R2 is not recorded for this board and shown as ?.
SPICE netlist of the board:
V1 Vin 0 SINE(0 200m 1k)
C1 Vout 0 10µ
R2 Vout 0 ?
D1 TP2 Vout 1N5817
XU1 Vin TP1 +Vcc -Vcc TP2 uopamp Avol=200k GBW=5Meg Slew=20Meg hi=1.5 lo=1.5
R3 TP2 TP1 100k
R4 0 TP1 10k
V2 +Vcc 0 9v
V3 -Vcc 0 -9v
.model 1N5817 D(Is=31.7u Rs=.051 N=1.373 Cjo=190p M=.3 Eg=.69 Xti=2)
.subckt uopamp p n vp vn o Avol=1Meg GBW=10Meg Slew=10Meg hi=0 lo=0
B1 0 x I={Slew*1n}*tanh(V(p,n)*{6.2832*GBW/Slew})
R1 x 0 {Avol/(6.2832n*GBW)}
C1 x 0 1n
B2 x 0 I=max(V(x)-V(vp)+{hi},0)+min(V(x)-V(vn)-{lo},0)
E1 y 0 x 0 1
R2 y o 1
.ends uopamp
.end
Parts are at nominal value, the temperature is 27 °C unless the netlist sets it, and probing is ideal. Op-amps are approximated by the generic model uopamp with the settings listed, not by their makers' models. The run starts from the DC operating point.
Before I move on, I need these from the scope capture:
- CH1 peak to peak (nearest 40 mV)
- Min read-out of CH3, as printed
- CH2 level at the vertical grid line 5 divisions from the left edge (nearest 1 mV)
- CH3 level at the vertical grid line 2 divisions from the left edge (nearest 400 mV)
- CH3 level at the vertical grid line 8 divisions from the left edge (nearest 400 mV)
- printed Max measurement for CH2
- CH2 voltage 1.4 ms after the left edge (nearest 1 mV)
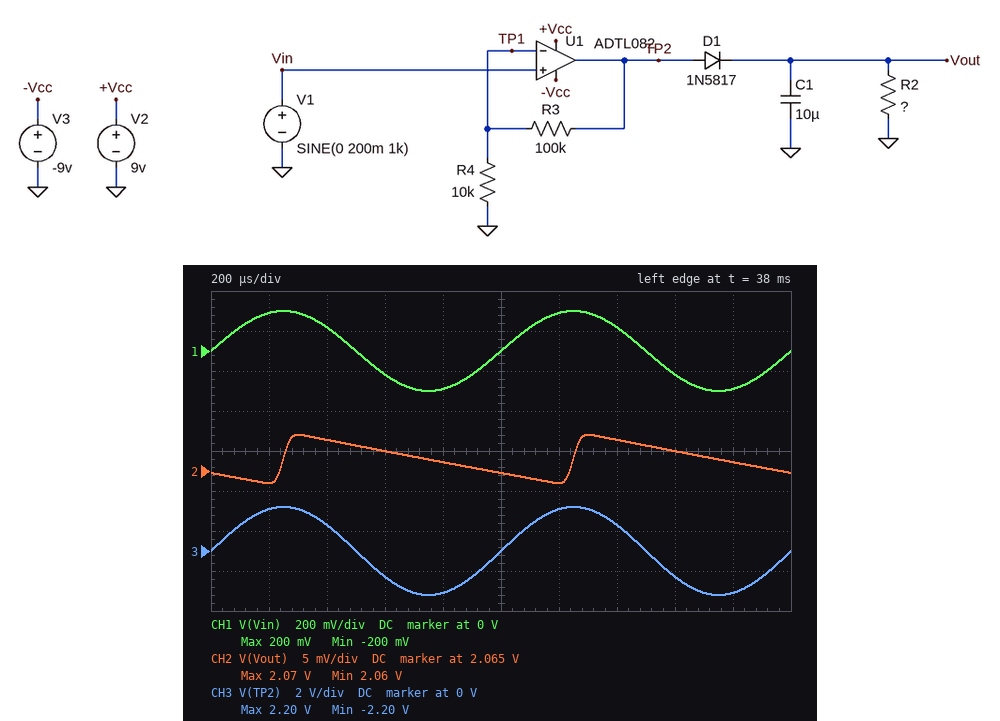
400 mV
-2.20 V
2.065 V
1.2 V
-1.2 V
2.07 V
2.069 V
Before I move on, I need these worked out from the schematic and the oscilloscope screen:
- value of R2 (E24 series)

56 kΩ
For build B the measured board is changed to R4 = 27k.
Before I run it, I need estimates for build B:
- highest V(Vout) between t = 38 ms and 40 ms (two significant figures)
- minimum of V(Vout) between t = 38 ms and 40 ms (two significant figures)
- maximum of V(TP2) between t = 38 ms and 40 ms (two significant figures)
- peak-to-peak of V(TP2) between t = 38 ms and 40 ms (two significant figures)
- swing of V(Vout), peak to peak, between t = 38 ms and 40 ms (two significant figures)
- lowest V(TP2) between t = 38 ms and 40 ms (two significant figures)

840 mV
830 mV
940 mV
1.9 V
3.9 mV
-940 mV
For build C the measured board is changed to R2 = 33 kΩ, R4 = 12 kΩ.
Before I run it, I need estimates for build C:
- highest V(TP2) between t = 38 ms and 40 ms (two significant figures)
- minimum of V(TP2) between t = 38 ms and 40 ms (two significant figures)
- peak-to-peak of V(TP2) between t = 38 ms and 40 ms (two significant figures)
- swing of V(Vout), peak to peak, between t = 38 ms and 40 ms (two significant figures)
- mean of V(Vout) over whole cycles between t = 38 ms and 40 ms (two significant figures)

1.9 V
-1.9 V
3.7 V
7.4 mV
1.7 V
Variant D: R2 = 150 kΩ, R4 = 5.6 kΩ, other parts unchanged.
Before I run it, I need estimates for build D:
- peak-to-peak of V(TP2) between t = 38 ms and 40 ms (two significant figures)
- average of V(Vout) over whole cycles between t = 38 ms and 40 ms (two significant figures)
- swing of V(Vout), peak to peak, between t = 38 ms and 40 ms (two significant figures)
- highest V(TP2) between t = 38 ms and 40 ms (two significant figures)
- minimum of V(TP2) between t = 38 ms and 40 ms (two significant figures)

7.5 V
3.6 V
5.1 mV
3.8 V
-3.8 V
